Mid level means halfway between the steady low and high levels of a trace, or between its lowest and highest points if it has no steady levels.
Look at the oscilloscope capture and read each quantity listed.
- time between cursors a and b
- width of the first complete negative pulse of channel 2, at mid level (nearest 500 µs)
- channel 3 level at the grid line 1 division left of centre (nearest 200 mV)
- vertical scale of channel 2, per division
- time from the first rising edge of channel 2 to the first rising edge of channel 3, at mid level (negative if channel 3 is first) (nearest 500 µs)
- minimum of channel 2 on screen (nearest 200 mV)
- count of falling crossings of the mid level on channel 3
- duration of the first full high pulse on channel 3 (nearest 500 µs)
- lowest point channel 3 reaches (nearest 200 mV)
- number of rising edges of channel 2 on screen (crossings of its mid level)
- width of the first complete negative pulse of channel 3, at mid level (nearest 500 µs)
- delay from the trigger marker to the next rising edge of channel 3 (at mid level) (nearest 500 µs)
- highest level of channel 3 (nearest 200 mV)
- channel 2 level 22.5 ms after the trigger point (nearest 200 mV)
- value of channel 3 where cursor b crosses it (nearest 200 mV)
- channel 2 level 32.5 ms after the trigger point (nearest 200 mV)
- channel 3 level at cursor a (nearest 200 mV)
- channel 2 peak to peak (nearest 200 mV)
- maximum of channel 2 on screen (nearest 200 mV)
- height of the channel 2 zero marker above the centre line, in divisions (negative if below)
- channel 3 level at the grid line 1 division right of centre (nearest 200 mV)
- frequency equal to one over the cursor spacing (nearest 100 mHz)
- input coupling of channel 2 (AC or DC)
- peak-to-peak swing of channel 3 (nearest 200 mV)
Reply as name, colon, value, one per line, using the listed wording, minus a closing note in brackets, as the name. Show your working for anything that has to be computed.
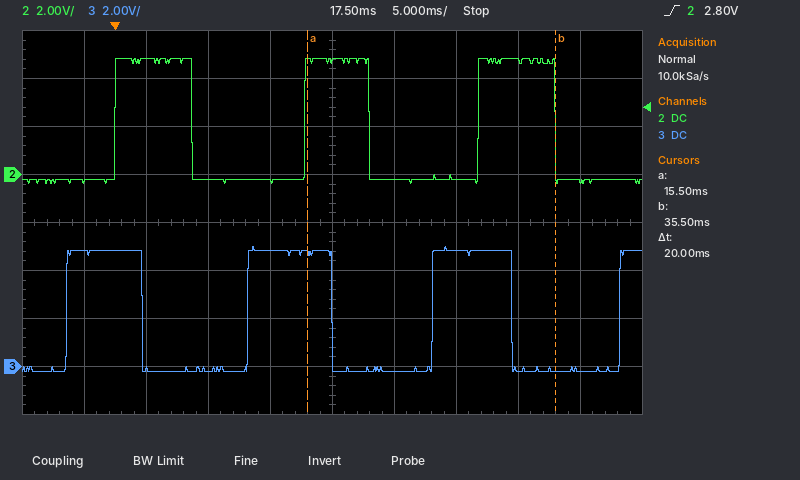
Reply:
time between cursors a and b: 20 ms
width of the first complete negative pulse of channel 2, at mid level: 9.0 ms
channel 3 level at the grid line 1 division left of centre: 4.8 V
vertical scale of channel 2, per division: 2 V
time from the first rising edge of channel 2 to the first rising edge of channel 3, at mid level (negative if channel 3 is first): -4.0 ms
minimum of channel 2 on screen: -400 mV
count of falling crossings of the mid level on channel 3: 3
duration of the first full high pulse on channel 3: 6.0 ms
lowest point channel 3 reaches: -200 mV
number of rising edges of channel 2 on screen: 3
width of the first complete negative pulse of channel 3, at mid level: 8.5 ms
delay from the trigger marker to the next rising edge of channel 3 (at mid level): 10.5 ms
highest level of channel 3: 5.0 V
channel 2 level 22.5 ms after the trigger point: -200 mV
value of channel 3 where cursor b crosses it: -200 mV
channel 2 level 32.5 ms after the trigger point: 4.8 V
channel 3 level at cursor a: 4.8 V
channel 2 peak to peak: 4.8 V − (-400 mV) = 5.2 V
maximum of channel 2 on screen: 4.8 V
height of the channel 2 zero marker above the centre line, in divisions: +1.0 div
channel 3 level at the grid line 1 division right of centre: -200 mV
frequency equal to one over the cursor spacing: 1 / 20 ms ≈ 50.0 Hz
input coupling of channel 2: DC
peak-to-peak swing of channel 3: 5.0 V − (-200 mV) = 5.2 V
